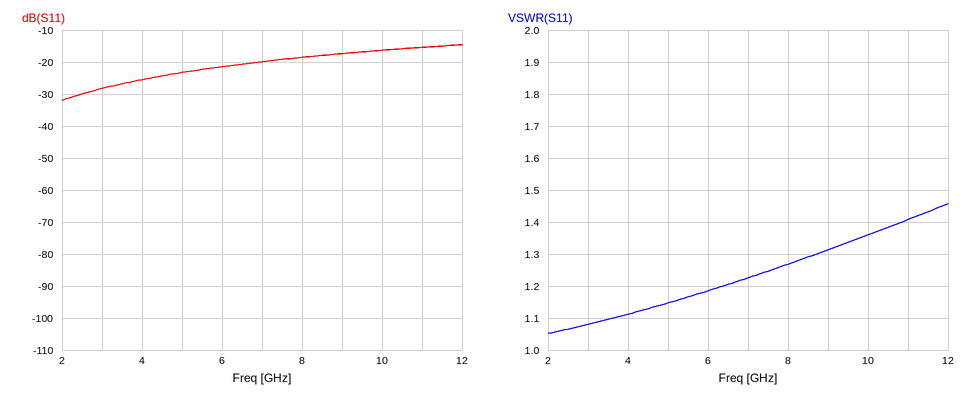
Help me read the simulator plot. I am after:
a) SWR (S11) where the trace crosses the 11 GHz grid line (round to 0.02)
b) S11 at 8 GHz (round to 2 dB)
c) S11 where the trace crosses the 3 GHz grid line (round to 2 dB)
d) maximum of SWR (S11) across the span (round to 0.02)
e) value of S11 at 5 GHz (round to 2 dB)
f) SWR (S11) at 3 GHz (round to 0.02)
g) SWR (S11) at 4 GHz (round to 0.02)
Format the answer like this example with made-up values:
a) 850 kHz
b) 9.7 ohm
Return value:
a) 1.40
b) -18 dB
c) -28 dB
d) 1.46
e) -24 dB
f) 1.08
g) 1.12
